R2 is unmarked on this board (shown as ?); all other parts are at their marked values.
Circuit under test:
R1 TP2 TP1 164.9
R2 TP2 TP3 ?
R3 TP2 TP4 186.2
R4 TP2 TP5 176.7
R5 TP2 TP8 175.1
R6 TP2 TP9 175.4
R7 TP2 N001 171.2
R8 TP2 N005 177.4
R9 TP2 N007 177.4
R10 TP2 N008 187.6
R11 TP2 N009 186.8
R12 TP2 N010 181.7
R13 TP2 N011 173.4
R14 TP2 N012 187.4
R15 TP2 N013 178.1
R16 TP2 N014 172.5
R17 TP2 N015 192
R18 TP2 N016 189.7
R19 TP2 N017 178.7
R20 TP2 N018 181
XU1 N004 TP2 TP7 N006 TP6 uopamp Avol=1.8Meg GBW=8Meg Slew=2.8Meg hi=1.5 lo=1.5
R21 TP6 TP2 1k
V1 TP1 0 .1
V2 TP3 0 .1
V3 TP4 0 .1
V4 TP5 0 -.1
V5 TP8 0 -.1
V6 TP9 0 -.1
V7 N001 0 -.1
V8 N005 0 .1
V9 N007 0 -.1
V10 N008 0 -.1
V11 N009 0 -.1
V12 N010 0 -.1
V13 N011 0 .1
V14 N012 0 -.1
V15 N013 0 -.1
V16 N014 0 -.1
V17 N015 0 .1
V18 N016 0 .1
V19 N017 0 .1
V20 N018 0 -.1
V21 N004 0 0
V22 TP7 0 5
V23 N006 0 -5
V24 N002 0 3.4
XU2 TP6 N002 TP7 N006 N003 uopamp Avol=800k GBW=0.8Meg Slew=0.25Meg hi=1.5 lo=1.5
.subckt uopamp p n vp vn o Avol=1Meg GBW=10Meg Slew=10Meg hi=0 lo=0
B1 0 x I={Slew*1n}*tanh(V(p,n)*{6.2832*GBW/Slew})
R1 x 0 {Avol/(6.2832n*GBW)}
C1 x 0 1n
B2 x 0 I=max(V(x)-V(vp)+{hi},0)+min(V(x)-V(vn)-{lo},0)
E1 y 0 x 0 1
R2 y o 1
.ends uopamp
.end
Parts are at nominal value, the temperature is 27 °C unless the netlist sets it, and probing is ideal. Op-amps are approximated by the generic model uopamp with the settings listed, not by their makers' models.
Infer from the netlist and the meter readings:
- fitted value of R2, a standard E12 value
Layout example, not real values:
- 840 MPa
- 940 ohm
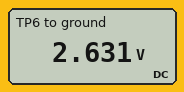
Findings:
- 560 Ω
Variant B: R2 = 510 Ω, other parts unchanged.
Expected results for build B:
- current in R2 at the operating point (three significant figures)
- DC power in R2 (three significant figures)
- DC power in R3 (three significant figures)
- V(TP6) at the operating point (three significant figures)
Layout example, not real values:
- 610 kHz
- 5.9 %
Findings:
- 196 µA
- 19.6 µW
- 53.7 µW
- 2.61 V
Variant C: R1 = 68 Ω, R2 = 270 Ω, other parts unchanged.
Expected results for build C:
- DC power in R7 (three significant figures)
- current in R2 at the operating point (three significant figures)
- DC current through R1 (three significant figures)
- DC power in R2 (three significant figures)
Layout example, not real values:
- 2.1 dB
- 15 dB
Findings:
- 58.4 µW
- 370 µA
- 1.47 mA
- 37.0 µW
